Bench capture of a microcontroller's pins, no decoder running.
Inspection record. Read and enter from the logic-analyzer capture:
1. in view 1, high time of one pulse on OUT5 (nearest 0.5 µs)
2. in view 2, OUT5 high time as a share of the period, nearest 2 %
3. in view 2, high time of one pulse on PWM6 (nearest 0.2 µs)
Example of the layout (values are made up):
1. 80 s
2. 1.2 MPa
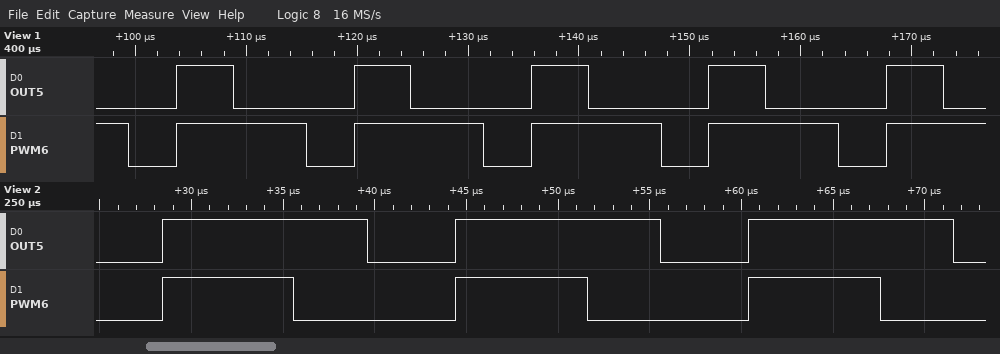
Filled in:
1. 5.0 µs
2. 70 %
3. 7.2 µs
